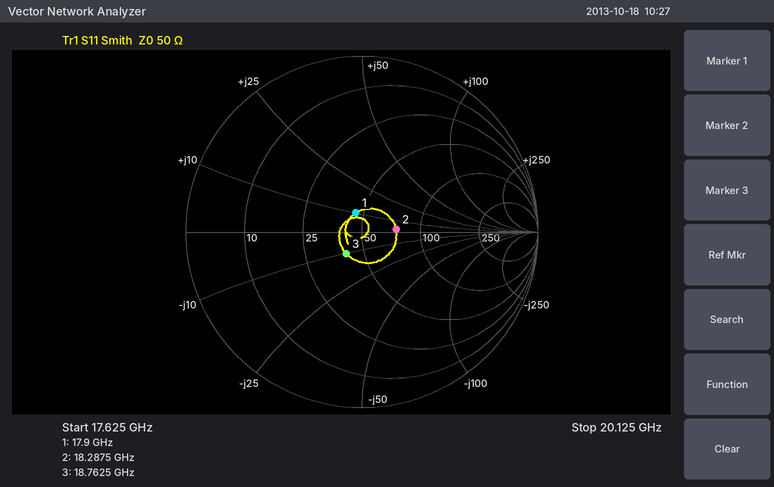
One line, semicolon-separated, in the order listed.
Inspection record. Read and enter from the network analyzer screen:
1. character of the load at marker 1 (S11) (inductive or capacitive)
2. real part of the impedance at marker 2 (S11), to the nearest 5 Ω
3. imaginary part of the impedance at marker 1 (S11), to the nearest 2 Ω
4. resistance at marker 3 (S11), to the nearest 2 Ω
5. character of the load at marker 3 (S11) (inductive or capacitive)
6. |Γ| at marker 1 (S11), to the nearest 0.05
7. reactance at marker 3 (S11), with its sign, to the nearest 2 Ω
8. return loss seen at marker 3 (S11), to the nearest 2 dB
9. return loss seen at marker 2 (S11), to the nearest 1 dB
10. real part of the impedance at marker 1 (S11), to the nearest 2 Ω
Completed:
inductive; 75 Ω; +10 Ω; 40 Ω; capacitive; 0.10; -10 Ω; 16 dB; 14 dB; 46 Ω
